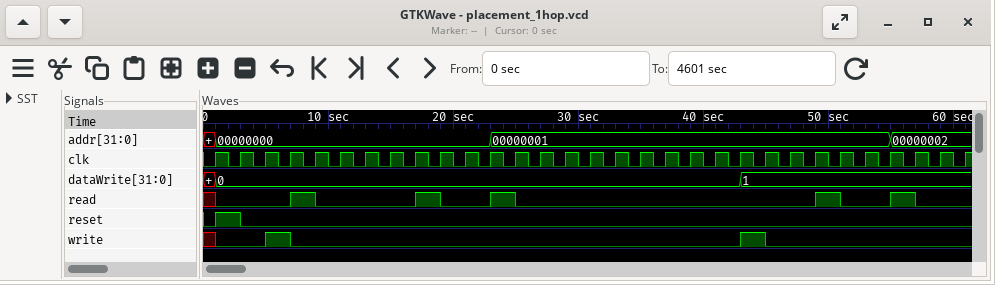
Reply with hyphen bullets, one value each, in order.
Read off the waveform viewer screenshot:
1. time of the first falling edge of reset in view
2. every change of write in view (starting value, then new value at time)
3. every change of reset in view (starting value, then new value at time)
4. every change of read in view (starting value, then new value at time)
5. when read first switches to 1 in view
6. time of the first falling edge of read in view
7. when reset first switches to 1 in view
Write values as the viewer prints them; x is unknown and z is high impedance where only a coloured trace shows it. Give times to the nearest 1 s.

- 3 s
- x, 0 at 1 s, 1 at 5 s, 0 at 7 s, 1 at 43 s, 0 at 45 s
- 0, 1 at 1 s, 0 at 3 s
- x, 0 at 1 s, 1 at 7 s, 0 at 9 s, 1 at 17 s, 0 at 19 s, 1 at 23 s, 0 at 25 s, 1 at 49 s, 0 at 51 s, 1 at 55 s, 0 at 57 s
- 7 s
- 9 s
- 1 s
